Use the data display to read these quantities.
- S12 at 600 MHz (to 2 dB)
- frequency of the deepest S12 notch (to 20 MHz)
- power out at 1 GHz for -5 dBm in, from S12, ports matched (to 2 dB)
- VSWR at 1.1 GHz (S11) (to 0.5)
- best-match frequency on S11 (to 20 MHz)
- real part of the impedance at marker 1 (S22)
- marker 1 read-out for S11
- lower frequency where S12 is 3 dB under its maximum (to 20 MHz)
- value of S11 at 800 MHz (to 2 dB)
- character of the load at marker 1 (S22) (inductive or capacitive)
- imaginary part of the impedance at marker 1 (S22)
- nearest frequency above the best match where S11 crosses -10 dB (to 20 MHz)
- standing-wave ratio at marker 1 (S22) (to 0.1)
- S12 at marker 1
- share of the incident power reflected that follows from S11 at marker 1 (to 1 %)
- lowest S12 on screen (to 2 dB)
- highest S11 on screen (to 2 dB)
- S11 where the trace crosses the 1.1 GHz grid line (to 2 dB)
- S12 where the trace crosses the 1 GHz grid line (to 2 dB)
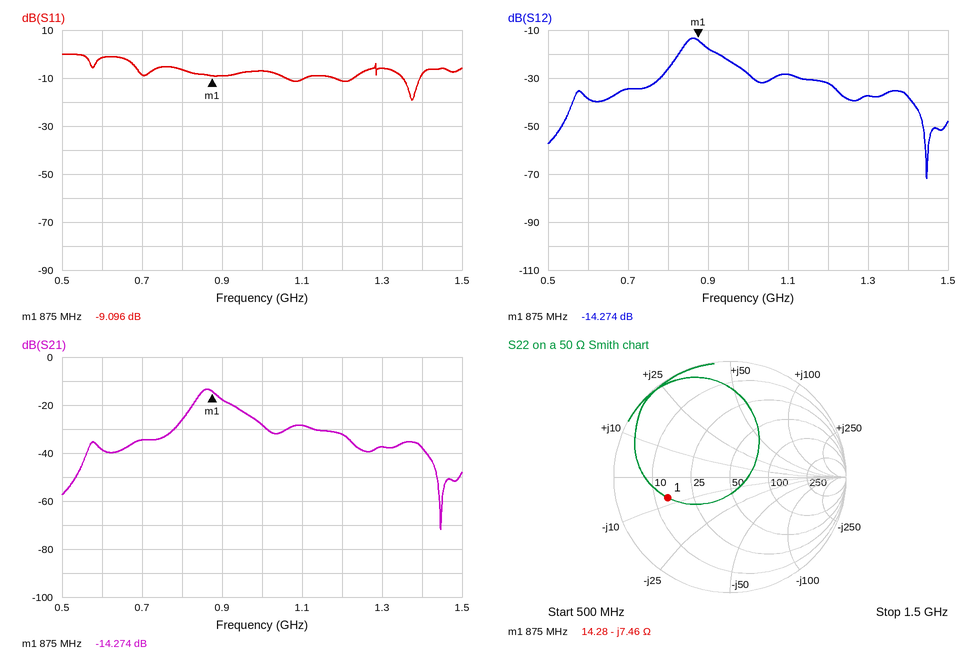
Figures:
-38 dB
1.44 GHz
-34 dBm
2.0
1.38 GHz
14.28 Ω
-9.096 dB
840 MHz
-6 dB
capacitive
-7.46 Ω
1.40 GHz
3.6
-14.274 dB
12 %
-72 dB
0 dB
-10 dB
-28 dB
